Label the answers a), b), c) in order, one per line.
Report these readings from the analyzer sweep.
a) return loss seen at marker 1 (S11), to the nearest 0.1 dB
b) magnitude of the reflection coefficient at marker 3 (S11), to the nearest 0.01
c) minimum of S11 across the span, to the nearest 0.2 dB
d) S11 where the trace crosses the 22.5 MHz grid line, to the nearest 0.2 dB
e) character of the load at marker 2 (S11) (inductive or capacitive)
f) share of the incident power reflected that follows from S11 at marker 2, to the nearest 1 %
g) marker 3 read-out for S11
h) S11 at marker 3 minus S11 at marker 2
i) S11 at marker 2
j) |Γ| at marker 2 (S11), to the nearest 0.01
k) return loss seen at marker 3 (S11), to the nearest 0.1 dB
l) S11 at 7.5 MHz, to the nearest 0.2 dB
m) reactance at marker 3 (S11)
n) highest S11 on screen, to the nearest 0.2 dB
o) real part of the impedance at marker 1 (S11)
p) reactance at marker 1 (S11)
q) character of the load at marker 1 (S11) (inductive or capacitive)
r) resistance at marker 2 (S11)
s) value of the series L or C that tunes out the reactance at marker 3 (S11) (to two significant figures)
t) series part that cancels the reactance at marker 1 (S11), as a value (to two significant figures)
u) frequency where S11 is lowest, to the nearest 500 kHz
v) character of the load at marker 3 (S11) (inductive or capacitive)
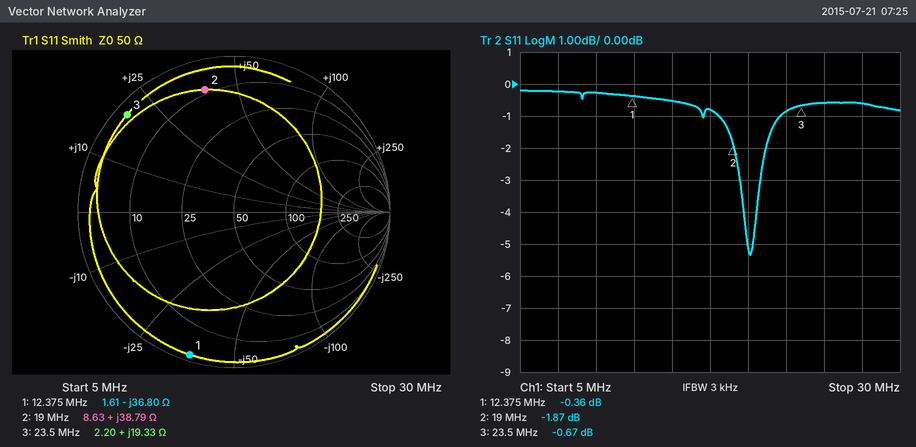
a) 0.4 dB
b) 0.93
c) -5.4 dB
d) -0.8 dB
e) inductive
f) 65 %
g) -0.67 dB
h) 1.20 dB
i) -1.87 dB
j) 0.81
k) 0.7 dB
l) -0.2 dB
m) +19.33 Ω
n) -0.2 dB
o) 1.61 Ω
p) -36.80 Ω
q) capacitive
r) 8.63 Ω
s) 350 pF
t) 470 nH
u) 20.0 MHz
v) inductive
